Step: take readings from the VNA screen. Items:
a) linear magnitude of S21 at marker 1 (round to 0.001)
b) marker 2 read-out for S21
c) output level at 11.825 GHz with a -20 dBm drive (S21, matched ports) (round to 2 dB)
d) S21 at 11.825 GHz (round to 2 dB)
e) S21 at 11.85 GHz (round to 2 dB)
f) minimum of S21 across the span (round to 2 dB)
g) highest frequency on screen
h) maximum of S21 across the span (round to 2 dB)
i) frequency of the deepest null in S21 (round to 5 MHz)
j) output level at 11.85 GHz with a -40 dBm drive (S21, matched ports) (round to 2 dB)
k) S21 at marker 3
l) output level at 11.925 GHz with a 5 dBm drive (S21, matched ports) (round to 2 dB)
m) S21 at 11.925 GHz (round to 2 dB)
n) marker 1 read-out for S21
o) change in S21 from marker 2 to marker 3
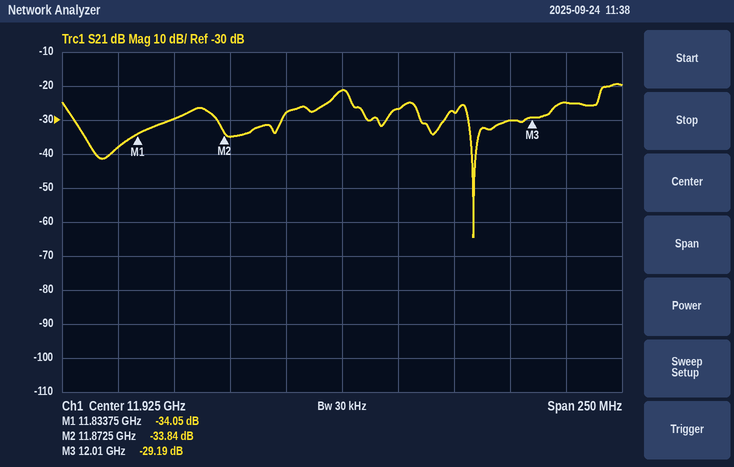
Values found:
0.020
-33.84 dB
-58 dBm
-38 dB
-30 dB
-64 dB
12.05 GHz
-20 dB
11.985 GHz
-70 dBm
-29.19 dB
-16 dBm
-22 dB
-34.05 dB
4.65 dB
